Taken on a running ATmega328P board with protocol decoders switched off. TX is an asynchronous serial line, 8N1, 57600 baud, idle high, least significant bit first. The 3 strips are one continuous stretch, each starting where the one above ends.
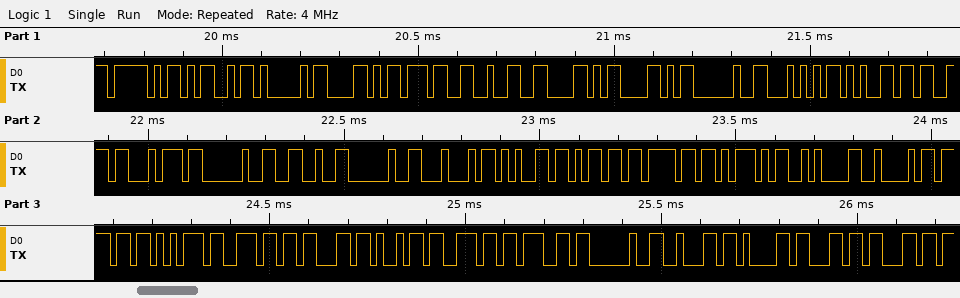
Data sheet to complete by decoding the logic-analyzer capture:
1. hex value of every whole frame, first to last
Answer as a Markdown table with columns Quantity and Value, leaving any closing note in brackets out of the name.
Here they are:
| Quantity | Value |
|---|---|
| hex value of every whole frame, first to last | 5F 4D 41 58 37 32 58 58 20 54 65 73 74 20 26 20 44 65 6D 6F 5D 0A 42 6F 75 6E 63 69 6E 67 20 62 61 6C 6C |
